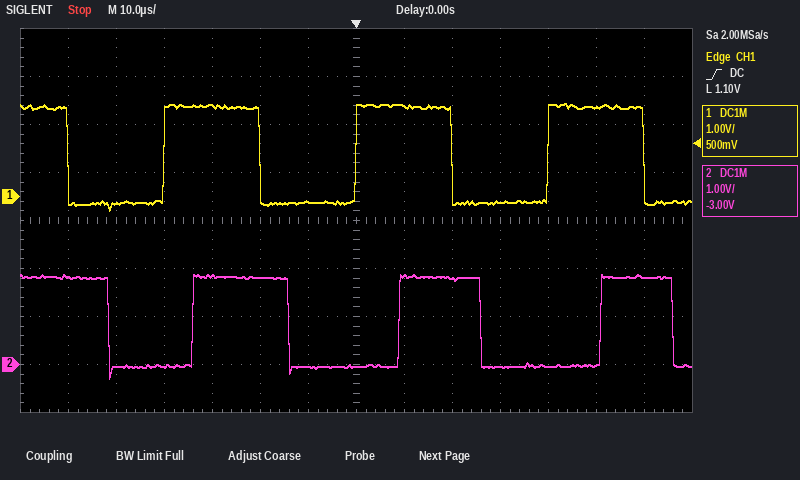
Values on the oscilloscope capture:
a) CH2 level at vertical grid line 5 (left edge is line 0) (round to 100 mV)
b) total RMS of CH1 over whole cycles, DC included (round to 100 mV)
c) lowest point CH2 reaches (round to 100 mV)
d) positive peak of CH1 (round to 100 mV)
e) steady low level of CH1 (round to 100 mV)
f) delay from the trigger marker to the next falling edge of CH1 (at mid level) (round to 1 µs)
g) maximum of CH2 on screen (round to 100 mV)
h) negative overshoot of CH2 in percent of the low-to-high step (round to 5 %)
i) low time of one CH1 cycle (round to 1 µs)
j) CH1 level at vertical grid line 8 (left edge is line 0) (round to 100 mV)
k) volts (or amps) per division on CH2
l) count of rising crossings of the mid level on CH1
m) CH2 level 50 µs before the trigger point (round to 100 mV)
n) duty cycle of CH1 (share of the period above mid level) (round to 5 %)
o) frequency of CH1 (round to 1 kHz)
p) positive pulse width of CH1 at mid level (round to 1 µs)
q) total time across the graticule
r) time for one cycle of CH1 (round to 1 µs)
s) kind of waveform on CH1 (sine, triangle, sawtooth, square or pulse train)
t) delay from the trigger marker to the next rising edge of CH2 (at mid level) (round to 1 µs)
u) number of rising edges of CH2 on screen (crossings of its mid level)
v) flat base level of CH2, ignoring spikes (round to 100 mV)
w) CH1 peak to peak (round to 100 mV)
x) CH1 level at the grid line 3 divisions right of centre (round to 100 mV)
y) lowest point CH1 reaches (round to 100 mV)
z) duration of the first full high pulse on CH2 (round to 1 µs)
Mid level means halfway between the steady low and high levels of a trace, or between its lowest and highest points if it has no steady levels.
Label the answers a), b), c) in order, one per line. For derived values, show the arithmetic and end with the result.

a) 1.8 V
b) √(0.5 × (1.9 V)² + 0.5 × (-100 mV)²) ≈ 1.3 V
c) -300 mV
d) 1.9 V
e) -100 mV
f) 20 µs
g) 1.9 V
h) 15 %
i) 20 µs
j) 1.9 V
k) 1 V
l) 3
m) 0.0 V
n) 20 µs / 40 µs ≈ 50 %
o) 1 / 40 µs ≈ 25 kHz
p) 20 µs
q) 140 µs
r) 40 µs
s) square
t) 9 µs
u) 3
v) 0.0 V
w) 1.9 V − (-300 mV) = 2.2 V
x) -100 mV
y) -300 mV
z) 20 µs
